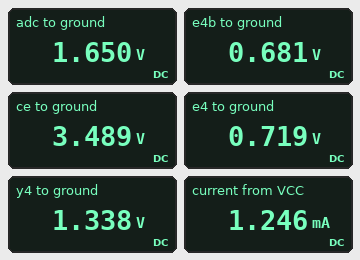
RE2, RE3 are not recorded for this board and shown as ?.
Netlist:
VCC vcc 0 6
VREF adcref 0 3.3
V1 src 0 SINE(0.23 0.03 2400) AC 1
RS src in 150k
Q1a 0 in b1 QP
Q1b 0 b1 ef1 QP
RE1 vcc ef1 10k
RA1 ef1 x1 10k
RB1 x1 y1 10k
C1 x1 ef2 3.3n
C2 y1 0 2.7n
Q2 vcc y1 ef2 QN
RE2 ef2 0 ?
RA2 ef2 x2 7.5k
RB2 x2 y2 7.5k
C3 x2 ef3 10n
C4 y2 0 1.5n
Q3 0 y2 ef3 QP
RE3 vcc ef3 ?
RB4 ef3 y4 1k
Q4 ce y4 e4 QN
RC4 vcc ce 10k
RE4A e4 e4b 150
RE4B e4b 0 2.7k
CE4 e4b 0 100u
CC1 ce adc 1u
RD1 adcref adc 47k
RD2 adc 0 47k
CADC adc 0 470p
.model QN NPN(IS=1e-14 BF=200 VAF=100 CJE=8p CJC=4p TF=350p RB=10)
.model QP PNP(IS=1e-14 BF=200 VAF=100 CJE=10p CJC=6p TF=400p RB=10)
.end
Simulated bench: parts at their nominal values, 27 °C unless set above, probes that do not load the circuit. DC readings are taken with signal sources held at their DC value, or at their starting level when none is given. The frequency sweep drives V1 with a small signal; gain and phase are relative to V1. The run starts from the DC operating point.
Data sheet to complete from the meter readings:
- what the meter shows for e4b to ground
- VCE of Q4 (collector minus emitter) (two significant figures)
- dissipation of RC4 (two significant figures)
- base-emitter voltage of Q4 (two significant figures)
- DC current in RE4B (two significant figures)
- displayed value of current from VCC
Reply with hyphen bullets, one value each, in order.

- 0.681 V
- 2.8 V
- 630 µW
- 620 mV
- 250 µA
- 1.246 mA
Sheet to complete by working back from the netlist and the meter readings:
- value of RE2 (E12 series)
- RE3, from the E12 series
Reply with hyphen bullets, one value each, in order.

- 2.2 kΩ
- 22 kΩ
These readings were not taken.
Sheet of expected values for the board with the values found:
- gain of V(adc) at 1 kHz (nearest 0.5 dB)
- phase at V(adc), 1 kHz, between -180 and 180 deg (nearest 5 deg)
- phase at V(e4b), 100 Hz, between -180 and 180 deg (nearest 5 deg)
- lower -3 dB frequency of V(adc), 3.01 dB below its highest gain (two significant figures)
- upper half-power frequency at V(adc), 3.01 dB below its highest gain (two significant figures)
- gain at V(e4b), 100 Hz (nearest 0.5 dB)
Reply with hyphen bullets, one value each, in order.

- 27.5 dB
- 150 deg
- -90 deg
- 8.9 Hz
- 5.0 kHz
- -25.0 dB
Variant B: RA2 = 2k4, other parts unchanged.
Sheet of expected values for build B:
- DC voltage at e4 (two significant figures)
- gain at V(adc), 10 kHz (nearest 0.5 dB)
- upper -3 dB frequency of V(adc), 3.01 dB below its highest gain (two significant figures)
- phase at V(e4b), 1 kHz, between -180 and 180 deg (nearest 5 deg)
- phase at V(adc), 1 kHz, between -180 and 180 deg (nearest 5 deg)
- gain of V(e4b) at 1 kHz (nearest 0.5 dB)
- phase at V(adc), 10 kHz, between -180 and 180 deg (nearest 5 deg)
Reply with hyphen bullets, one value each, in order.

- 710 mV
- 13.5 dB
- 4.4 kHz
- -115 deg
- 155 deg
- -45.5 dB
- -55 deg
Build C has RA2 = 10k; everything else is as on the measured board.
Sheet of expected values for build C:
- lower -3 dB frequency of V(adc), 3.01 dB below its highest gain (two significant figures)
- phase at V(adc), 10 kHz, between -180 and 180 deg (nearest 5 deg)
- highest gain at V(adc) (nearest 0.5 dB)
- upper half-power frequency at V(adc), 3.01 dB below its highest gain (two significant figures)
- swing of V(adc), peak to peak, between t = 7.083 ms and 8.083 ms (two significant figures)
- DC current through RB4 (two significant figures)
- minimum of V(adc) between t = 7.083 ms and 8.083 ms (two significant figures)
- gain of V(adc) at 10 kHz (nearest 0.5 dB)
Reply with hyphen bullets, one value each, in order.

- 9.2 Hz
- -105 deg
- 28.0 dB
- 4.6 kHz
- 1.5 V
- 1.2 µA
- 870 mV
- 2.0 dB
